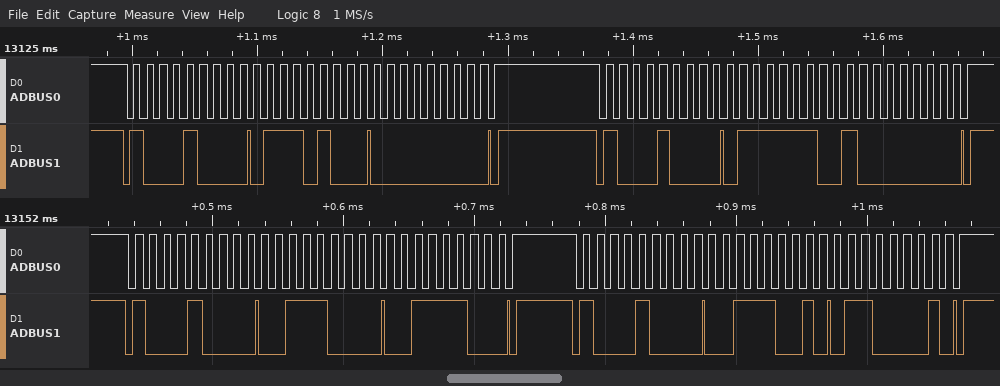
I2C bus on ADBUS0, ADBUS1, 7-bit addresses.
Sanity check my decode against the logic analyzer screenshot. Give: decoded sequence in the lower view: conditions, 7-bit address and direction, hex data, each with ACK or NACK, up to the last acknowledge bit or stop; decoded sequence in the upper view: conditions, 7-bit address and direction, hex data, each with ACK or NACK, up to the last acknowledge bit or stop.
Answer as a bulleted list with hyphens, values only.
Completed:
- start, address 44 write ACK, 38 ACK, 3C ACK, stop, start, address 44 write ACK, 39 ACK, 61 ACK, stop
- start, address 44 write ACK, 74 ACK, 00 ACK, stop, start, address 44 write ACK, 7E ACK, 80 ACK, stop
